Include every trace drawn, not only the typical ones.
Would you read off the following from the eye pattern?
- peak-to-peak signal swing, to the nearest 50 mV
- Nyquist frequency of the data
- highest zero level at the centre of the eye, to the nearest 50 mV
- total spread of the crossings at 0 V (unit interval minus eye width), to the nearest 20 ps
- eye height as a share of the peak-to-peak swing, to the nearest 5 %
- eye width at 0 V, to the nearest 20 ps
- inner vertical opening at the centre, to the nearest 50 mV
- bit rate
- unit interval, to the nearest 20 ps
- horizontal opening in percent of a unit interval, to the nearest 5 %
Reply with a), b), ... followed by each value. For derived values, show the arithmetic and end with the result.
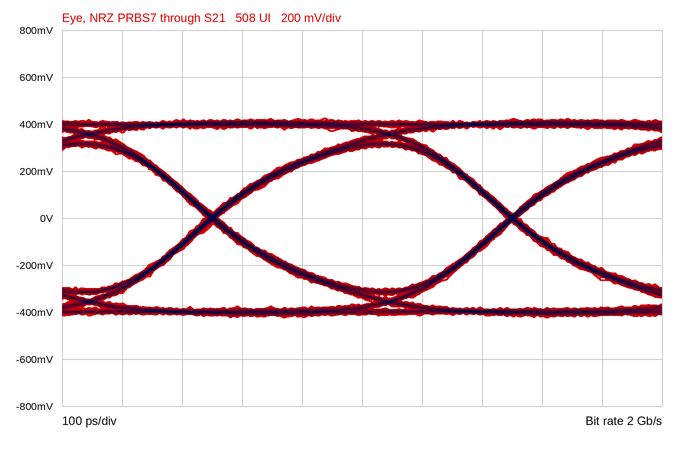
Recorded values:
a) 850 mV
b) 1 GHz
c) -300 mV
d) 20 ps
e) 600 mV / 850 mV ≈ 70.6 %, so 70 % to the nearest 5 %
f) 480 ps
g) 600 mV
h) 2 Gb/s
i) 500 ps
j) 480 ps / 500 ps ≈ 96.0 %, so 95 % to the nearest 5 %
